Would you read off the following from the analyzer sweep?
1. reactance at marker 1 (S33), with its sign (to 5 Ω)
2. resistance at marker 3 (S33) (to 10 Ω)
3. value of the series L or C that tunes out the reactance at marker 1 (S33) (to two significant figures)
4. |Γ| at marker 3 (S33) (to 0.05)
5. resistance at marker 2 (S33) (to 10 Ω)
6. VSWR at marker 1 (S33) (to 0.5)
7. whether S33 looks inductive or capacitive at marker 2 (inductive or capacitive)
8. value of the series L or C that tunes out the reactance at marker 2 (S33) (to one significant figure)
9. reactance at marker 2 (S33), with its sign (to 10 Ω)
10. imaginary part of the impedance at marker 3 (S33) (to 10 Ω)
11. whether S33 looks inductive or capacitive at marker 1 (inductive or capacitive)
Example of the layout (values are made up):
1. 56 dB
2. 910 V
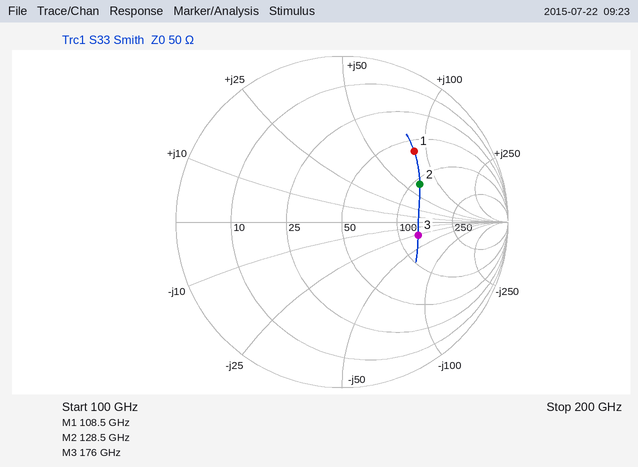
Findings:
1. +85 Ω
2. 130 Ω
3. 17 fF
4. 0.45
5. 110 Ω
6. 4.0
7. inductive
8. 20 fF
9. +70 Ω
10. -30 Ω
11. inductive
